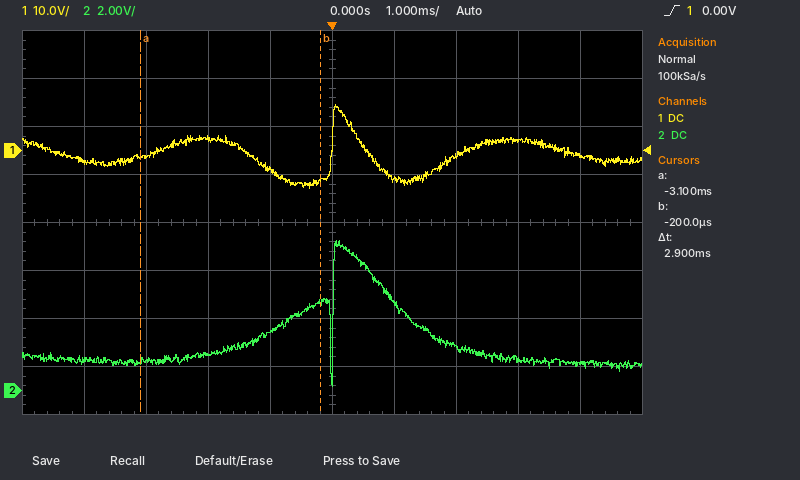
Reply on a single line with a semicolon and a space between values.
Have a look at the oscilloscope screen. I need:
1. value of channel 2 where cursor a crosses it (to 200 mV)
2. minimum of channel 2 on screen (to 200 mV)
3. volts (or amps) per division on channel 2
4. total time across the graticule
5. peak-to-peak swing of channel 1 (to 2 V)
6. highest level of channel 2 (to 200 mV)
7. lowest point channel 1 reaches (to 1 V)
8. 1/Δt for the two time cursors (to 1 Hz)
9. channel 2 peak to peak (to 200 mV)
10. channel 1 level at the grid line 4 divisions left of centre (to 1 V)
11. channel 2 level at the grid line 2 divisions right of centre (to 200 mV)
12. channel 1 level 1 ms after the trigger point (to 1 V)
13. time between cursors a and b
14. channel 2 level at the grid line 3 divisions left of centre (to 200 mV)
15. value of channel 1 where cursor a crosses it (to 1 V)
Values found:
1.2 V; 200 mV; 2 V; 10 ms; 18 V; 6.2 V; -8 V; 345 Hz; 6.0 V; -2 V; 1.8 V; -6 V; 2.9 ms; 1.2 V; -1 V
